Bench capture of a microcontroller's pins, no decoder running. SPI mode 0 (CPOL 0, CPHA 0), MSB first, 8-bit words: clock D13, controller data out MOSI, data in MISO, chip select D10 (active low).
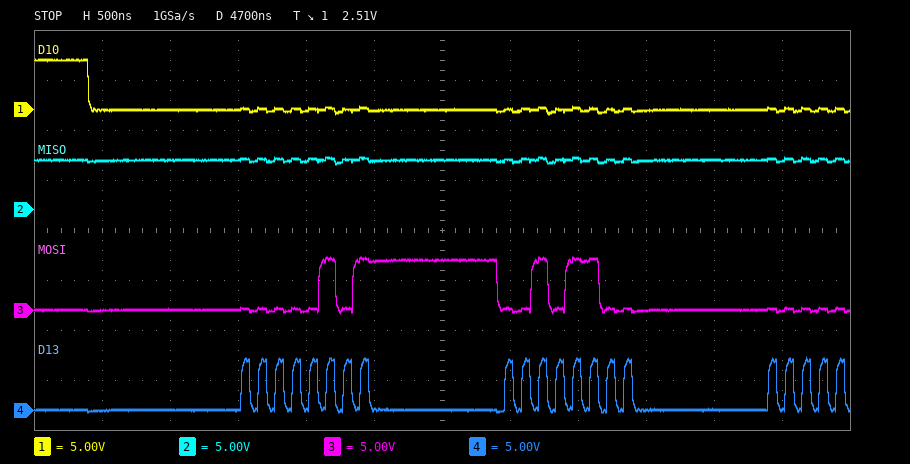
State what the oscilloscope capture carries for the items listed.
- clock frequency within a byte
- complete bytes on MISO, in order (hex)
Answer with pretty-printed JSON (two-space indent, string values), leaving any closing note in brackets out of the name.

{
  "clock frequency within a byte": "8 MHz",
  "complete bytes on MISO, in order": "0xFF 0xFF"
}
